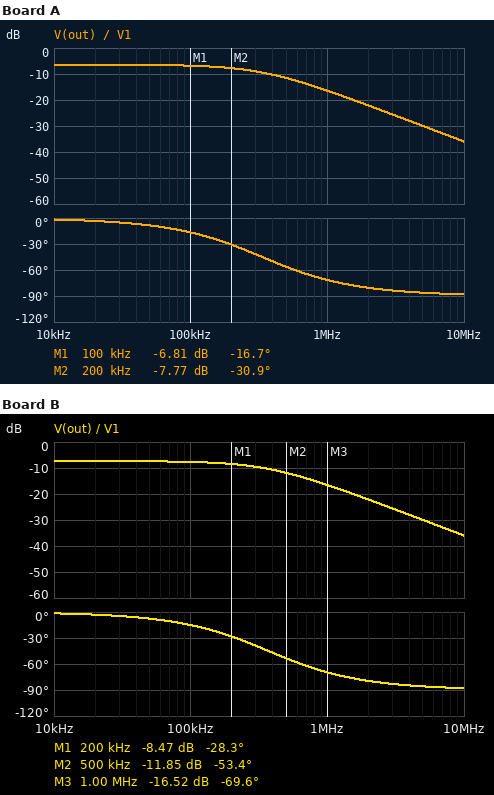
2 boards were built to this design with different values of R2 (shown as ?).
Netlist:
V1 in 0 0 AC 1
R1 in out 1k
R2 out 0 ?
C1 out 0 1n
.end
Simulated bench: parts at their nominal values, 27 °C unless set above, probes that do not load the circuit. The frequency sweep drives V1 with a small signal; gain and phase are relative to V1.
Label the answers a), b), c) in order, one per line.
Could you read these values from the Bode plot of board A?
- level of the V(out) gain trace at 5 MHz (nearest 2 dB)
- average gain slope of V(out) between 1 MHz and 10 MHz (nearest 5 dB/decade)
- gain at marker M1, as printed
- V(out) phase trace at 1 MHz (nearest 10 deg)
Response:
a) -30 dB
b) -20 dB/decade
c) -6.81 dB
d) -70 deg
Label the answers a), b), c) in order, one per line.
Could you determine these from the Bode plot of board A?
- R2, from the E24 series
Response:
a) 910 Ω
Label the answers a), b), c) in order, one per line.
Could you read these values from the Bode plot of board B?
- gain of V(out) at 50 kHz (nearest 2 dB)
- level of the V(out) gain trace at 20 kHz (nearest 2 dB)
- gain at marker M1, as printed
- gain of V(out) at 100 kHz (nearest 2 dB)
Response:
a) -8 dB
b) -8 dB
c) -8.47 dB
d) -8 dB
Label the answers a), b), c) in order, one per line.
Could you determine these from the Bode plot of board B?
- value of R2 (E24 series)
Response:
a) 750 Ω
